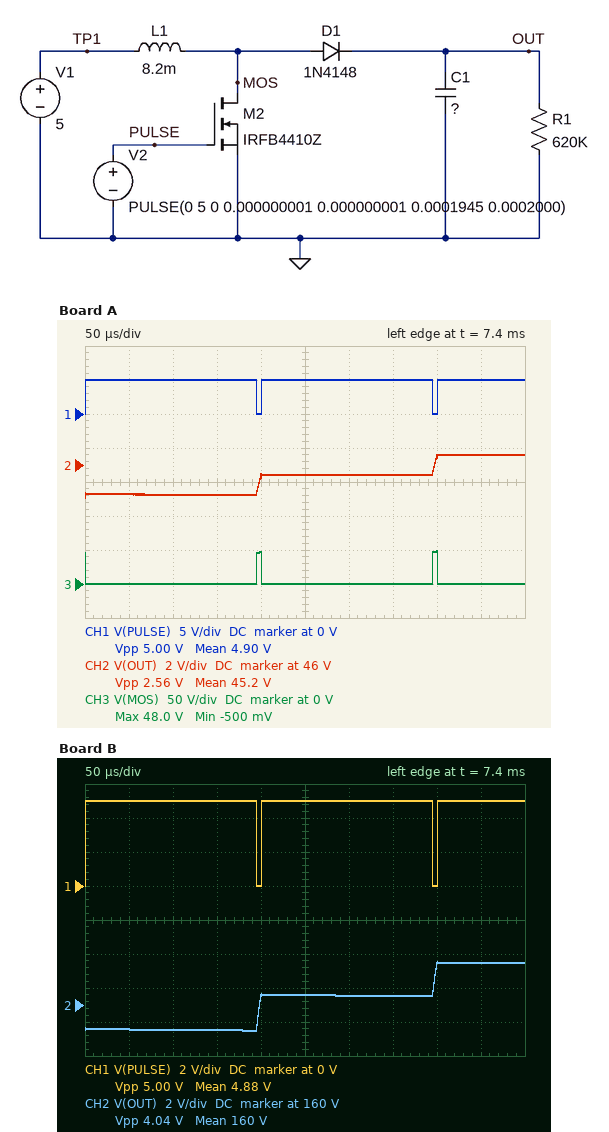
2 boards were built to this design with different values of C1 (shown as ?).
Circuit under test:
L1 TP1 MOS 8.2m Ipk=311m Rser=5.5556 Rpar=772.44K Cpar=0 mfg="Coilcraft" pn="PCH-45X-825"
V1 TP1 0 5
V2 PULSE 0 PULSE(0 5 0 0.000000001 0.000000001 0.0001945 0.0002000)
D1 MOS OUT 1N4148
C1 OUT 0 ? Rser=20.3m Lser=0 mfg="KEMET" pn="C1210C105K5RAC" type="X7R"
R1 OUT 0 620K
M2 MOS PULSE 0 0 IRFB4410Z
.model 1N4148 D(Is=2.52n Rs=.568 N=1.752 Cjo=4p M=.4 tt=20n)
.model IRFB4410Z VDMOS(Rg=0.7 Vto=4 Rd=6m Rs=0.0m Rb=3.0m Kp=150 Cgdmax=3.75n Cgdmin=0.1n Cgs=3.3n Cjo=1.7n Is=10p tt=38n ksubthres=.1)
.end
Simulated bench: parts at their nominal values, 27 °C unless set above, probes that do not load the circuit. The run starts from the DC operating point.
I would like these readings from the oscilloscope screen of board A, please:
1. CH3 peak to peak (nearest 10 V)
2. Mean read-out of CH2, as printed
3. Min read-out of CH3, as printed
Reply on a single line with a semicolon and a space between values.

50 V; 45.2 V; -500 mV
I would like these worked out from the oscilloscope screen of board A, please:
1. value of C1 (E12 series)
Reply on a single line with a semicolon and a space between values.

3.3 µF
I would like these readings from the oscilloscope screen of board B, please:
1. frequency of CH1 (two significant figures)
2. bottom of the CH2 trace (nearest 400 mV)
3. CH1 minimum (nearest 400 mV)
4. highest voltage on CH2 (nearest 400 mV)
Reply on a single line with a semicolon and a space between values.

5.0 kHz; 158.4 V; 0 V; 162.4 V
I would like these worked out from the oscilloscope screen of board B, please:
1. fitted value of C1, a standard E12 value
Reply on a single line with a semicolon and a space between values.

560 nF
